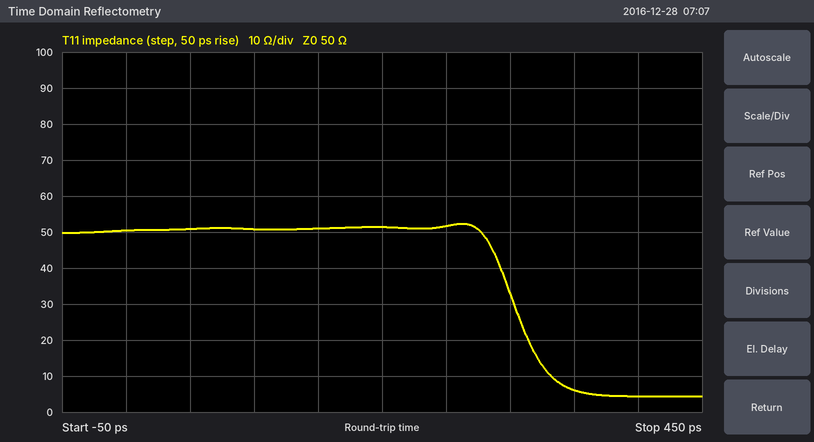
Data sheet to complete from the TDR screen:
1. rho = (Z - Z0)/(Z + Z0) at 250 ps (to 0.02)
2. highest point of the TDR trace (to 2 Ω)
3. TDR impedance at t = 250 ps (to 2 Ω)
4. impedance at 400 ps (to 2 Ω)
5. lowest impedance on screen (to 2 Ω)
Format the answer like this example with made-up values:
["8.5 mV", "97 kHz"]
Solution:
["+0.02", "52 Ω", "52 Ω", "4 Ω", "4 Ω"]
